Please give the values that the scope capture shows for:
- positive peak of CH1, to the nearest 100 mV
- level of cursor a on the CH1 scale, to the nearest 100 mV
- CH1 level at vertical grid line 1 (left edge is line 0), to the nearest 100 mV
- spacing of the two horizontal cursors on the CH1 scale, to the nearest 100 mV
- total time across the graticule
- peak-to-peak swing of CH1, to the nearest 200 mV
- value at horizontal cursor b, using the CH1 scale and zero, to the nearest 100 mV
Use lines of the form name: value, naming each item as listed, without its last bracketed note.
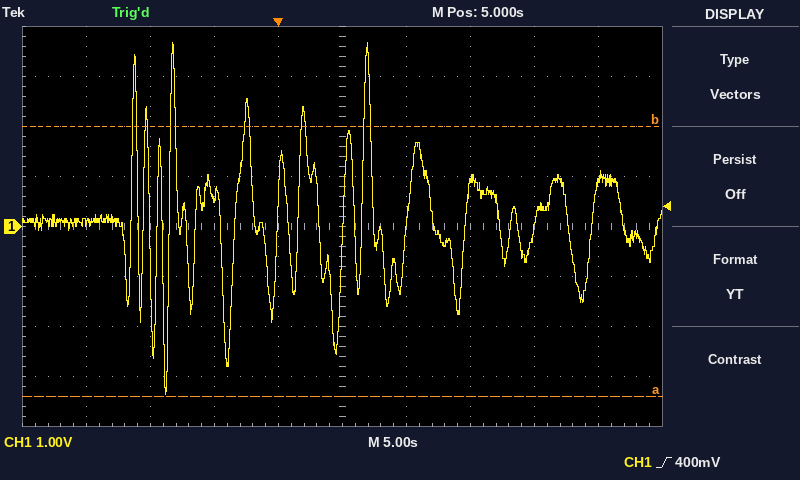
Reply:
positive peak of CH1, to the nearest 100 mV: 3.7 V
level of cursor a on the CH1 scale, to the nearest 100 mV: -3.4 V
CH1 level at vertical grid line 1 (left edge is line 0), to the nearest 100 mV: 100 mV
spacing of the two horizontal cursors on the CH1 scale, to the nearest 100 mV: 5.4 V
total time across the graticule: 50 s
peak-to-peak swing of CH1, to the nearest 200 mV: 7.0 V
value at horizontal cursor b, using the CH1 scale and zero, to the nearest 100 mV: 2.0 V
